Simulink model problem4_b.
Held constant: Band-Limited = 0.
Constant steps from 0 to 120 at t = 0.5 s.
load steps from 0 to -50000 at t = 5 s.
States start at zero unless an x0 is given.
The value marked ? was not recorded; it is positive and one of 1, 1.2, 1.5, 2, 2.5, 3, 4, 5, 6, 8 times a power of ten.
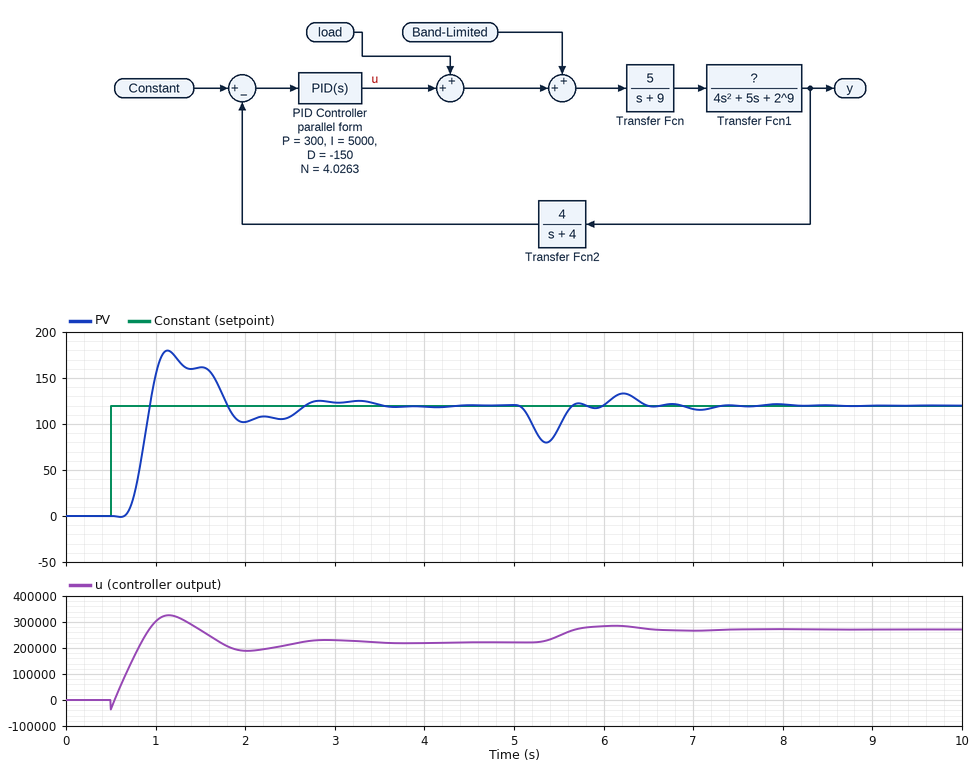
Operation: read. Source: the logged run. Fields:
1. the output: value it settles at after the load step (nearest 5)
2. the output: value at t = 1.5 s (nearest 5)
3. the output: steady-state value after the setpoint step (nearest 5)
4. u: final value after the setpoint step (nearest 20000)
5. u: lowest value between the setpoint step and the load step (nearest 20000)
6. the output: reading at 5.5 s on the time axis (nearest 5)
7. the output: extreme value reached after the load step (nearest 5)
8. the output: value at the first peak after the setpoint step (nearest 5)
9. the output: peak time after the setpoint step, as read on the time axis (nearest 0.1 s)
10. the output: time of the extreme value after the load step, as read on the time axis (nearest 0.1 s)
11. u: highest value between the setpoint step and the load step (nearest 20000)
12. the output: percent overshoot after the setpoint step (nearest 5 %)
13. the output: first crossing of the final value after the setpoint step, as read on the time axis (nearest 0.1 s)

120
160
120
220000
-40000
95
80
180
1.1 s
5.4 s
320000
50 %
0.9 s
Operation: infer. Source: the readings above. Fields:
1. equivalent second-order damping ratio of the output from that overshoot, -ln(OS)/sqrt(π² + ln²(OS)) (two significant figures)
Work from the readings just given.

0.22
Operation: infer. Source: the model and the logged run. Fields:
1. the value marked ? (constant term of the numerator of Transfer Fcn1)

0.5
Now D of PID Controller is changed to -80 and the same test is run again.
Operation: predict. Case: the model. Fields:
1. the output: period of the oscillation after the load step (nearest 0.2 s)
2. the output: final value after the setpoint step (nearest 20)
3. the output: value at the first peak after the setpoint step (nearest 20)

0.6 s
120
160
